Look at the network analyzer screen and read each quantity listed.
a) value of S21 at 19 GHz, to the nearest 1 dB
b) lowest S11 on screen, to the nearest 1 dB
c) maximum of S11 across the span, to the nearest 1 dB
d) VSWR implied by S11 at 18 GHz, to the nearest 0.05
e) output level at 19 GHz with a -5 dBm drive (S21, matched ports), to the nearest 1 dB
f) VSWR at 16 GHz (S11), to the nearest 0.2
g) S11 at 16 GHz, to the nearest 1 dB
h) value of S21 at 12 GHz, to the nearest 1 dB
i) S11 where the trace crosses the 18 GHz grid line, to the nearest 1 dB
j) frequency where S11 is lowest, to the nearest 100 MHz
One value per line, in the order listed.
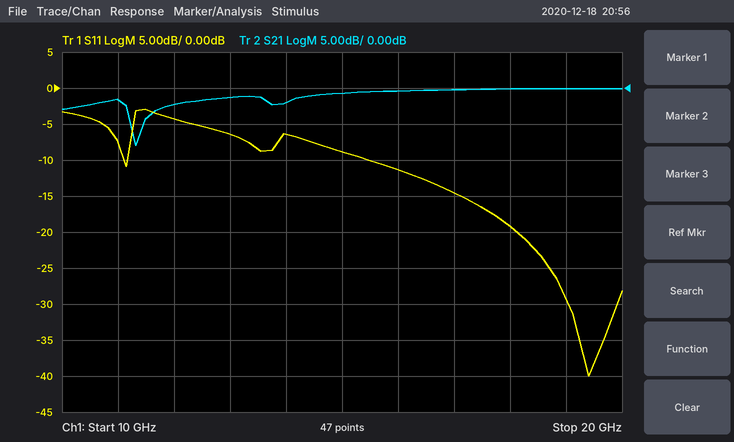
0 dB
-40 dB
-3 dB
1.25
-5 dBm
1.8
-11 dB
-2 dB
-19 dB
19.4 GHz
